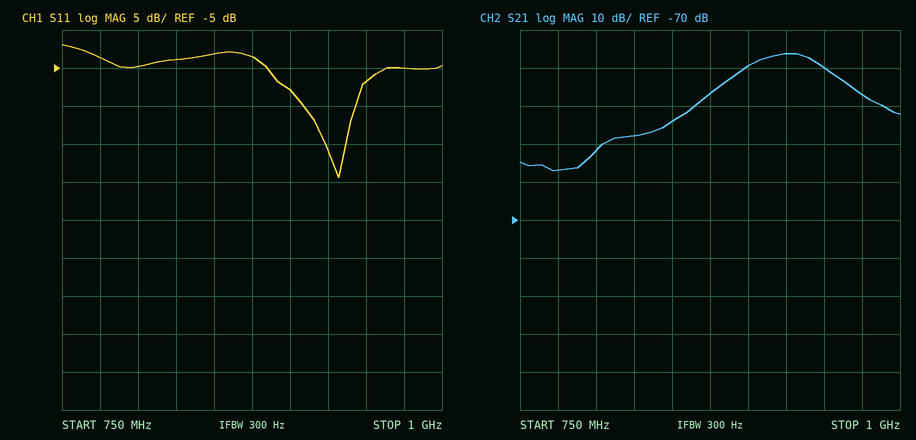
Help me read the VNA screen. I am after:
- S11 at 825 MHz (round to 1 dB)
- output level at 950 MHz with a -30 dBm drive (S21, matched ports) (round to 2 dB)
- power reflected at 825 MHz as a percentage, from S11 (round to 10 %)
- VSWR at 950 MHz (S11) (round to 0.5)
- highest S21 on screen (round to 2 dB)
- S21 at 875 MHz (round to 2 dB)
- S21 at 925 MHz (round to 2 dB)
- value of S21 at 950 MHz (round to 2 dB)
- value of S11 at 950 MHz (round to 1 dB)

-4 dB
-60 dBm
40 %
2.5
-26 dB
-36 dB
-26 dB
-30 dB
-7 dB
